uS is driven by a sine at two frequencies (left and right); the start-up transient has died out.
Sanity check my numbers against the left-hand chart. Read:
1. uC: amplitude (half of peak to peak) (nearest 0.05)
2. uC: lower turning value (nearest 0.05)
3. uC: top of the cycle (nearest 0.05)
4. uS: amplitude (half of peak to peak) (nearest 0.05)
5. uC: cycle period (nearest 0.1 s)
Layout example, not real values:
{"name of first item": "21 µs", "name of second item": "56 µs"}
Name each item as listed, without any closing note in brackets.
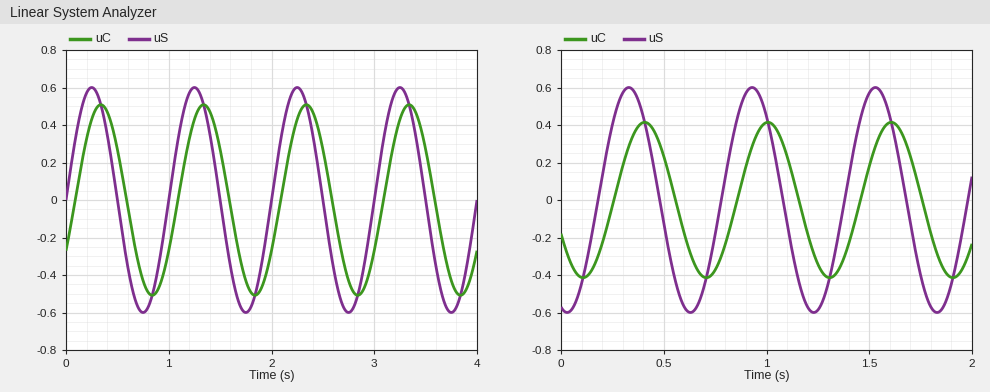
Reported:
{"uC: amplitude (half of peak to peak)": "0.50", "uC: lower turning value": "-0.50", "uC: top of the cycle": "0.50", "uS: amplitude (half of peak to peak)": "0.60", "uC: cycle period": "1.0 s"}
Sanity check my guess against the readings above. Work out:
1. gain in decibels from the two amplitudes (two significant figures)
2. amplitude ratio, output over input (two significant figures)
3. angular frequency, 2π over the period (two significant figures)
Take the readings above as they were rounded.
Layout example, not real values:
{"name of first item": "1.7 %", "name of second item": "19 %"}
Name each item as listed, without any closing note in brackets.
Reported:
{"gain in decibels from the two amplitudes": "-1.6 dB", "amplitude ratio, output over input": "0.83", "angular frequency, 2π over the period": "6.3 rad/s"}
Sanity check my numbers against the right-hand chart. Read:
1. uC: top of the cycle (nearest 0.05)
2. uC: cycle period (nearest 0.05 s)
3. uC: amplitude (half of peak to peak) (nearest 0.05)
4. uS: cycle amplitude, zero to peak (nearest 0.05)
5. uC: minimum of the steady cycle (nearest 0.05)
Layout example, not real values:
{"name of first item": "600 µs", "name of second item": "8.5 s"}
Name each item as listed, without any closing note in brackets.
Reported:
{"uC: top of the cycle": "0.40", "uC: cycle period": "0.60 s", "uC: amplitude (half of peak to peak)": "0.40", "uS: cycle amplitude, zero to peak": "0.60", "uC: minimum of the steady cycle": "-0.40"}
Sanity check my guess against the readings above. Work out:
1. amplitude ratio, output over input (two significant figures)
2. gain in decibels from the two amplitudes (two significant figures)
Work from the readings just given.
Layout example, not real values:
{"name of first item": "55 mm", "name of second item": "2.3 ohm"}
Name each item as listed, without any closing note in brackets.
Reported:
{"amplitude ratio, output over input": "0.67", "gain in decibels from the two amplitudes": "-3.5 dB"}
